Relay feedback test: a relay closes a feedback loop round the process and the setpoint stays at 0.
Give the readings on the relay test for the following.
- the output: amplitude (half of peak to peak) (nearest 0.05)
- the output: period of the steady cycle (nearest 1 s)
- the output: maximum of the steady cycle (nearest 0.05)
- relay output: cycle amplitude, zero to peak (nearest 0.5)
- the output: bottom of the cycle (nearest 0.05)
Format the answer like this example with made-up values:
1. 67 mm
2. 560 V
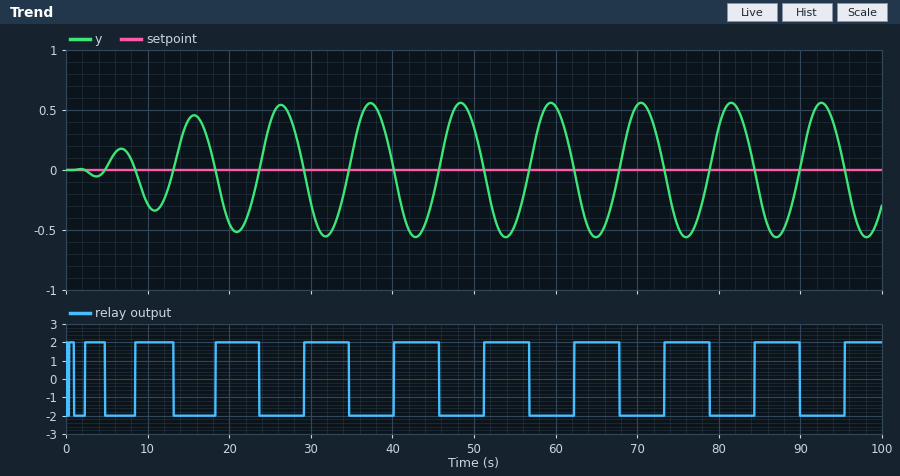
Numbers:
1. 0.55
2. 11 s
3. 0.55
4. 2.0
5. -0.55
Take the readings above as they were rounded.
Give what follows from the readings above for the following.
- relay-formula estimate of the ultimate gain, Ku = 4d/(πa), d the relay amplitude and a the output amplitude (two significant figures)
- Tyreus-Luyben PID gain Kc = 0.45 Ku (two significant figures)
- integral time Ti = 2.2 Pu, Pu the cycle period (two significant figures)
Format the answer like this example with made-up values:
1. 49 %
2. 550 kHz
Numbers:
1. 4.6
2. 2.1
3. 24 s
